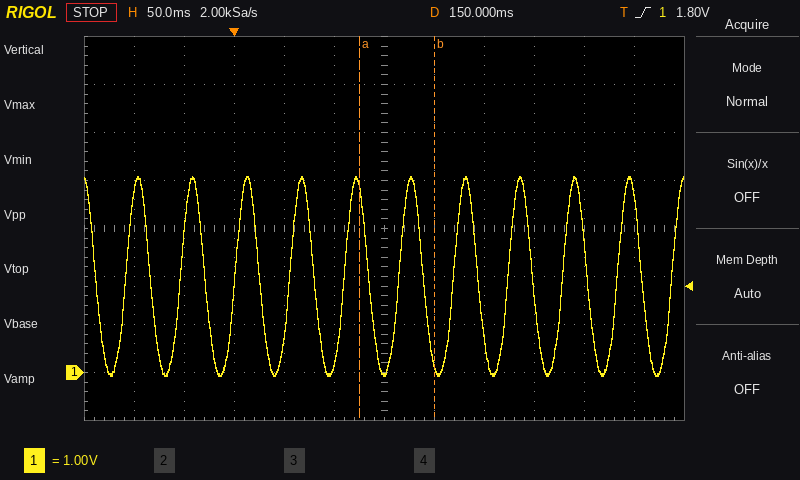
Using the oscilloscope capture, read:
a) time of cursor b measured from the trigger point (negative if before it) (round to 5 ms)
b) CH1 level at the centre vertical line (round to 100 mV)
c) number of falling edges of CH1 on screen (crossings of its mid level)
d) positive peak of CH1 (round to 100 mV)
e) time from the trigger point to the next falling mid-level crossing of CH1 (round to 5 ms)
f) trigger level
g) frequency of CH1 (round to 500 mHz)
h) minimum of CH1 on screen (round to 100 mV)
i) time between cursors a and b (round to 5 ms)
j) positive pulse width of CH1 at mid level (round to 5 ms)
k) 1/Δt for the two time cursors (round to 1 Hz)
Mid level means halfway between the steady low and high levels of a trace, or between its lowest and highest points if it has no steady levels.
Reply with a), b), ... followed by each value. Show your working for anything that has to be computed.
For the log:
a) +200 ms
b) 0.0 V
c) 11
d) 4.1 V
e) 25 ms
f) 1.80 V
g) 18.5 Hz
h) -100 mV
i) 75 ms
j) 25 ms
k) 1 / 75 ms ≈ 13 Hz
